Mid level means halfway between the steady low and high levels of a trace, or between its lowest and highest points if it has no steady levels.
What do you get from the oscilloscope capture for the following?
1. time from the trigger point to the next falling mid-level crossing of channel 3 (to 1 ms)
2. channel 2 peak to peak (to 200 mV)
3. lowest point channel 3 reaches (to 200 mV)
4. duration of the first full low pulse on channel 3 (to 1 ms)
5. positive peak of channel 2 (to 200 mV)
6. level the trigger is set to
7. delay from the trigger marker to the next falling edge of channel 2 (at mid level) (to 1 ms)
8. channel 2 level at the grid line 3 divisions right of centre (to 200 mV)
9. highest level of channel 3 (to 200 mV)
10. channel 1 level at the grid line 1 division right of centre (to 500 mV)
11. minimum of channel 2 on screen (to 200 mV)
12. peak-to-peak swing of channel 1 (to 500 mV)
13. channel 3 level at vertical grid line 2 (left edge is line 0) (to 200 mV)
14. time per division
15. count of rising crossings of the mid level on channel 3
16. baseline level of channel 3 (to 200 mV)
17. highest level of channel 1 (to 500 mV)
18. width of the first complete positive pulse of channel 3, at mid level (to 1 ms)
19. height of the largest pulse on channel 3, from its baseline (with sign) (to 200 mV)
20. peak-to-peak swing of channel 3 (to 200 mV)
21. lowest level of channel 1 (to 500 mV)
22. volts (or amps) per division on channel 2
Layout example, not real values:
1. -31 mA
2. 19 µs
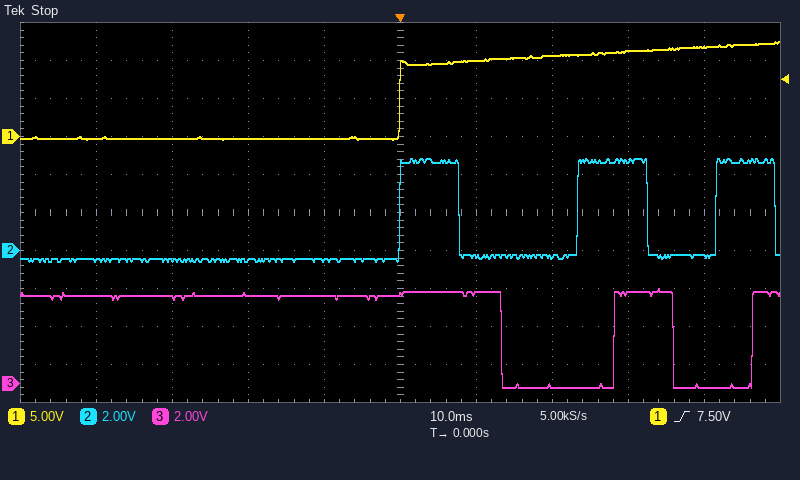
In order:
1. 13 ms
2. 5.4 V
3. -200 mV
4. 15 ms
5. 4.8 V
6. 7.50 V
7. 8 ms
8. 4.8 V
9. 5.0 V
10. 10.0 V
11. -600 mV
12. 13.0 V
13. 4.6 V
14. 10 ms
15. 2
16. 4.6 V
17. 12.5 V
18. 8 ms
19. -4.8 V
20. 5.2 V
21. -500 mV
22. 2 V
